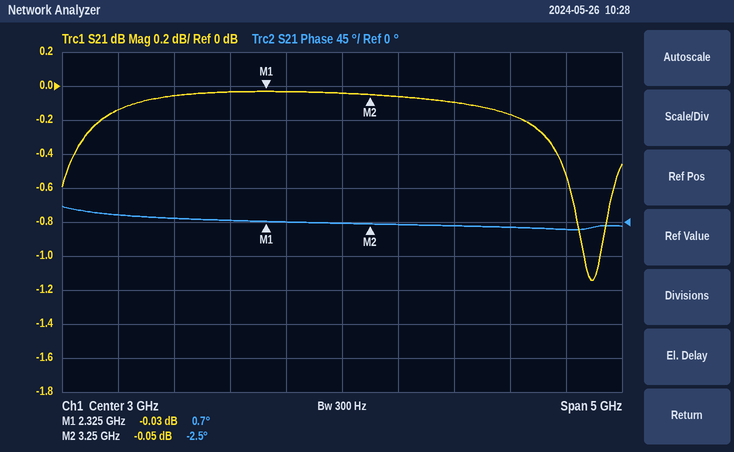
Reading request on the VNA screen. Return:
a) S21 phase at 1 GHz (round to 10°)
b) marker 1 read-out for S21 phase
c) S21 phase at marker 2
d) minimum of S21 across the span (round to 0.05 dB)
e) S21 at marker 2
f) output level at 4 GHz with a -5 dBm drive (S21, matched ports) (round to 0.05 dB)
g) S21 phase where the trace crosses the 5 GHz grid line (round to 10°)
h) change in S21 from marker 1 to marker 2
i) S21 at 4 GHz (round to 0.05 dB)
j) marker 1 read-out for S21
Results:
10°
0.7°
-2.5°
-1.15 dB
-0.05 dB
-5.10 dBm
-10°
-0.02 dB
-0.10 dB
-0.03 dB
